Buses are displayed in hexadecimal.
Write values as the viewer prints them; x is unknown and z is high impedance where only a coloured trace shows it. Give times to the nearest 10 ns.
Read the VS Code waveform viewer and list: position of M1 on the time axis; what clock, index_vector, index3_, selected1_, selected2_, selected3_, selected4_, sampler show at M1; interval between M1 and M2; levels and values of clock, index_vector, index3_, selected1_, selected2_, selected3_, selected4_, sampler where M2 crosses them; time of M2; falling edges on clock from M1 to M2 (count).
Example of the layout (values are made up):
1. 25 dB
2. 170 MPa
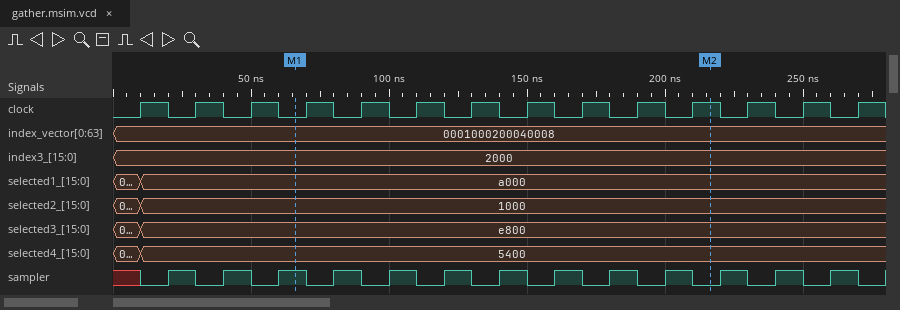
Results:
1. 70 ns
2. clock=0, index_vector=0001000200040008, index3_=2000, selected1_=a000, selected2_=1000, selected3_=e800, selected4_=5400, sampler=1
3. 150 ns
4. clock=1, index_vector=0001000200040008, index3_=2000, selected1_=a000, selected2_=1000, selected3_=e800, selected4_=5400, sampler=0
5. 220 ns
6. 7
